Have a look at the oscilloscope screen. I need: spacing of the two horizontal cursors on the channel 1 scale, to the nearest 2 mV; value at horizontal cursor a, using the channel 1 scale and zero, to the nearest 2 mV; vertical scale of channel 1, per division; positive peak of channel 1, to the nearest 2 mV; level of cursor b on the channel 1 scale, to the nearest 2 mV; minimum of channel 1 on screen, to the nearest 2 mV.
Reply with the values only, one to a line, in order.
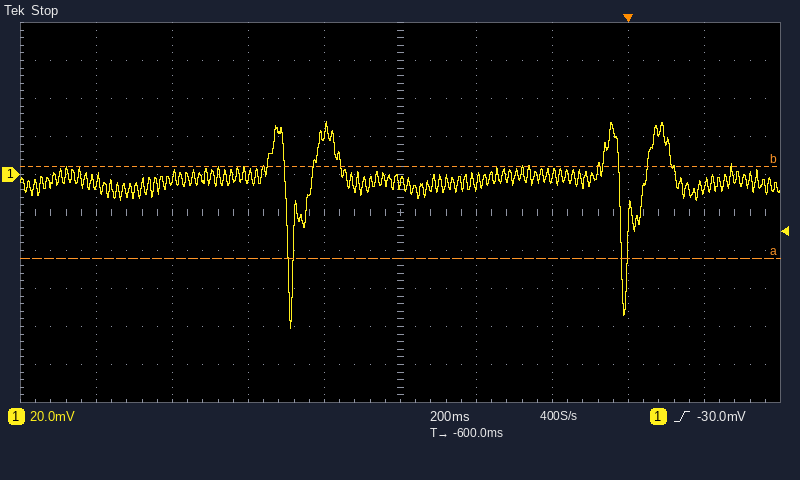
48 mV
-44 mV
20 mV
28 mV
4 mV
-82 mV
